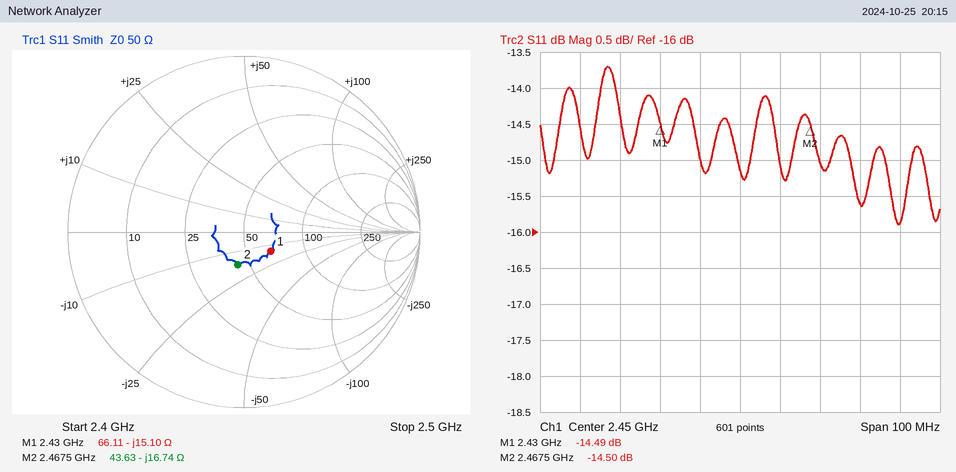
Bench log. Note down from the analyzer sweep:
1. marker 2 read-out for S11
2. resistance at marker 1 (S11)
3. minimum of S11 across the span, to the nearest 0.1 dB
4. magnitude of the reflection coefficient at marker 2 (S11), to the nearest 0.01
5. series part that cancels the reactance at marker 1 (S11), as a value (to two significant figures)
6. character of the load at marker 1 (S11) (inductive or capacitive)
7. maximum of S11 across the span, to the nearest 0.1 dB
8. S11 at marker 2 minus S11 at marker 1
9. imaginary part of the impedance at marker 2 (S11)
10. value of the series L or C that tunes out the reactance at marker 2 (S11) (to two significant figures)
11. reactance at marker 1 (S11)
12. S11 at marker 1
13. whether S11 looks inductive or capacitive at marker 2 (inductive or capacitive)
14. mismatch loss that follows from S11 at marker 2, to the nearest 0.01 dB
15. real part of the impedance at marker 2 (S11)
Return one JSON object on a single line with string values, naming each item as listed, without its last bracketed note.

{"marker 2 read-out for S11": "-14.50 dB", "resistance at marker 1": "66.11 Ω", "minimum of S11 across the span, to the nearest 0.1 dB": "-15.9 dB", "magnitude of the reflection coefficient at marker 2 (S11), to the nearest 0.01": "0.19", "series part that cancels the reactance at marker 1 (S11), as a value": "990 pH", "character of the load at marker 1 (S11)": "capacitive", "maximum of S11 across the span, to the nearest 0.1 dB": "-13.7 dB", "S11 at marker 2 minus S11 at marker 1": "-0.01 dB", "imaginary part of the impedance at marker 2": "-16.74 Ω", "value of the series L or C that tunes out the reactance at marker 2 (S11)": "1.1 nH", "reactance at marker 1": "-15.10 Ω", "S11 at marker 1": "-14.49 dB", "whether S11 looks inductive or capacitive at marker 2": "capacitive", "mismatch loss that follows from S11 at marker 2, to the nearest 0.01 dB": "0.16 dB", "real part of the impedance at marker 2": "43.63 Ω"}
